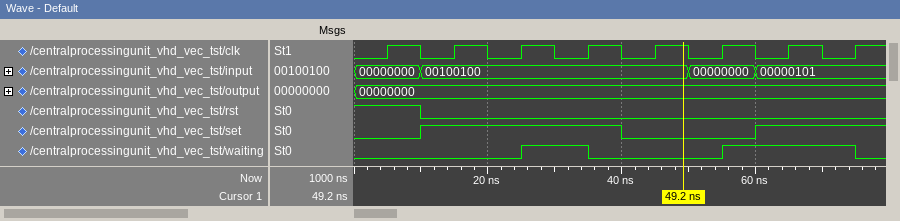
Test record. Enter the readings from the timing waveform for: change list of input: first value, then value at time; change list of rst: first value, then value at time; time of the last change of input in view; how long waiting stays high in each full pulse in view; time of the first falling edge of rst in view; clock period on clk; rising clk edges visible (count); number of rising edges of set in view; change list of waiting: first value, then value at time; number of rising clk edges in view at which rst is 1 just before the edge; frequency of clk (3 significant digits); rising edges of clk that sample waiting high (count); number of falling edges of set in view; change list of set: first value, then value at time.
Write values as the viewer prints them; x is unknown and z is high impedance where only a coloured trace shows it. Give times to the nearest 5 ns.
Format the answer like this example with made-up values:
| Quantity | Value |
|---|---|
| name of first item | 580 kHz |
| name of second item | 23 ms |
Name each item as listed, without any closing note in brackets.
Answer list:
| Quantity | Value |
|---|---|
| change list of input: first value, then value at time | 00000000, 00100100 at 10 ns, 00000000 at 50 ns, 00000101 at 60 ns |
| change list of rst: first value, then value at time | 1, 0 at 10 ns |
| time of the last change of input in view | 60 ns |
| how long waiting stays high in each full pulse in view | 10 ns, 20 ns |
| time of the first falling edge of rst in view | 10 ns |
| clock period on clk | 10 ns |
| rising clk edges visible | 8 |
| number of rising edges of set in view | 2 |
| change list of waiting: first value, then value at time | 0, 1 at 25 ns, 0 at 35 ns, 1 at 55 ns, 0 at 75 ns |
| number of rising clk edges in view at which rst is 1 just before the edge | 1 |
| frequency of clk | 100 MHz |
| rising edges of clk that sample waiting high | 3 |
| number of falling edges of set in view | 1 |
| change list of set: first value, then value at time | 0, 1 at 10 ns, 0 at 40 ns, 1 at 60 ns |
